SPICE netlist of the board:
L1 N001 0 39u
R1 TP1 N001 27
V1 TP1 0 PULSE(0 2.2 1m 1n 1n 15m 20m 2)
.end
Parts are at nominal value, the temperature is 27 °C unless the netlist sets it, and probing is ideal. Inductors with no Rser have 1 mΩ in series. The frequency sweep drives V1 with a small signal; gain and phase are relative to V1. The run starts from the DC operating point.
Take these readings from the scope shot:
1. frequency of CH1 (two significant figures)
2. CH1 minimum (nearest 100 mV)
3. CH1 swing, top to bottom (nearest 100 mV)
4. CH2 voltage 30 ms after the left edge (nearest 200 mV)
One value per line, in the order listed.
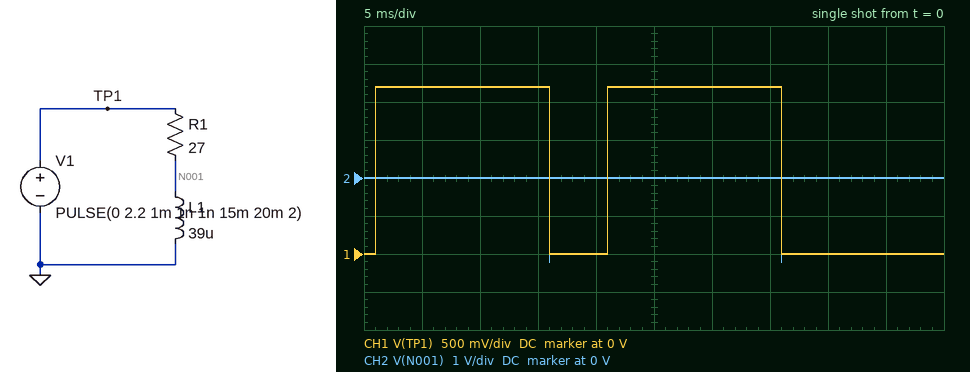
50 Hz
0 V
2.2 V
0 V
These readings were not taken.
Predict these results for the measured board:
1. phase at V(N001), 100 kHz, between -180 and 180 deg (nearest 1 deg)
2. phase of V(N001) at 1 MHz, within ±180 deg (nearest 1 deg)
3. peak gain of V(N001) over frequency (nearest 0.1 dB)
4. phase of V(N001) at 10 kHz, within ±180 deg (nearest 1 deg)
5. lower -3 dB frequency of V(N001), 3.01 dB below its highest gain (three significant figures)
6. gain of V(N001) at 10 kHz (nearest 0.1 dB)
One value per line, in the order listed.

48 deg
6 deg
0 dB
85 deg
110 kHz
-20.9 dB
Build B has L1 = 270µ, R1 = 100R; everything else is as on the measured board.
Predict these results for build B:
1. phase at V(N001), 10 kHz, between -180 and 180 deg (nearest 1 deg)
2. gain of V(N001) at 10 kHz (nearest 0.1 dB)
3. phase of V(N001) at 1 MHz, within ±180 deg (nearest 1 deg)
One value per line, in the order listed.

80 deg
-15.5 dB
3 deg
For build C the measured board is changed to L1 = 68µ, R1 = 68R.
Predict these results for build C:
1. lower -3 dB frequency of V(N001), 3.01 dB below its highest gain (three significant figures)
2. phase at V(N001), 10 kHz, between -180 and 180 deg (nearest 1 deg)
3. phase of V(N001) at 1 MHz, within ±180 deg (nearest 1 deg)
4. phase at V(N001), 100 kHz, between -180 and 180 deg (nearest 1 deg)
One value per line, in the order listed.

159 kHz
86 deg
9 deg
58 deg
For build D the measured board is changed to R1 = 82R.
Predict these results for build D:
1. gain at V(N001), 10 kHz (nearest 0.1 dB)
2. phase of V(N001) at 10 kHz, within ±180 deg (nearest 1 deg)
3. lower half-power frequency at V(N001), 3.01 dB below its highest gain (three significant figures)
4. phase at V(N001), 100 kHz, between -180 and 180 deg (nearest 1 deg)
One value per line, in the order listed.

-30.5 dB
88 deg
335 kHz
73 deg
